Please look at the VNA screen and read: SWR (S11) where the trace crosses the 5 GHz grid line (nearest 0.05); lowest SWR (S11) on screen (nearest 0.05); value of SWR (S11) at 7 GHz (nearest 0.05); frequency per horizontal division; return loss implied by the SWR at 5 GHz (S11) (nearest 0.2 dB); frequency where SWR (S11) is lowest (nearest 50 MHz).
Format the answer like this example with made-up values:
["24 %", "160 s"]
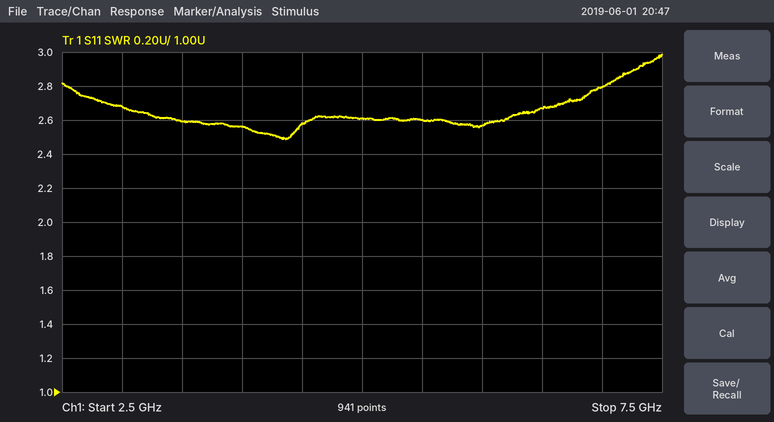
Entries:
["2.60", "2.50", "2.80", "500 MHz", "7.0 dB", "4.35 GHz"]
